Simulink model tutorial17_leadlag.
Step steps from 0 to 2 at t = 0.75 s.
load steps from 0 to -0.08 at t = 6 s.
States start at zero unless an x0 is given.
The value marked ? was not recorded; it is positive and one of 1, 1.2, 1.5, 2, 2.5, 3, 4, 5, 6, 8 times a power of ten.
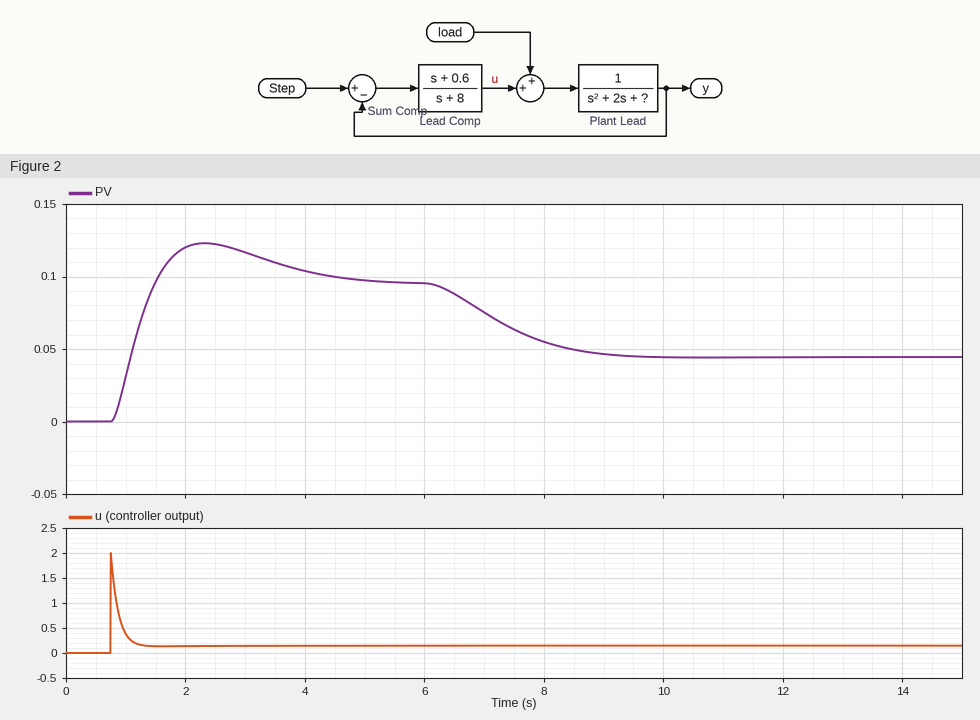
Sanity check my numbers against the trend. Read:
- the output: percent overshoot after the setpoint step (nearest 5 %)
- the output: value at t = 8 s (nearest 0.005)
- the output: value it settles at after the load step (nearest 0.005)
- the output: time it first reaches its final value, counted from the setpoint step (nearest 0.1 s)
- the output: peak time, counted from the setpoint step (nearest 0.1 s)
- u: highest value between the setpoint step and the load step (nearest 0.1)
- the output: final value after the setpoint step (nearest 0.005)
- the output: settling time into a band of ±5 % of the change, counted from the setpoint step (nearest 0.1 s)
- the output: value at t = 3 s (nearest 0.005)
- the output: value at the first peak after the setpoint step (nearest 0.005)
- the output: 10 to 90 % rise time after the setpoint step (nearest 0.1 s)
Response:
30 %
0.055
0.045
0.7 s
1.6 s
2.0
0.095
3.7 s
0.115
0.125
0.5 s
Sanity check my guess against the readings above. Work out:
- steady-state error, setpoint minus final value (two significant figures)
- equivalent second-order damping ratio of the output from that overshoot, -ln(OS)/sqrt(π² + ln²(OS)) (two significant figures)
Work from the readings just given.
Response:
1.9
0.36
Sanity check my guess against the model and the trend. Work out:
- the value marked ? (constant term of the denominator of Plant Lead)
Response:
1.5
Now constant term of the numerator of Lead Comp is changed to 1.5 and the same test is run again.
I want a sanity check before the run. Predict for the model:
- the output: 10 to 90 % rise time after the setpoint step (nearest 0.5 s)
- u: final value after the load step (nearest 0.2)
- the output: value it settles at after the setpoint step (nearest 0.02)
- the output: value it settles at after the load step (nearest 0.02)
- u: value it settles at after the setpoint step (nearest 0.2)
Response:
1.5 s
0.4
0.22
0.18
0.4
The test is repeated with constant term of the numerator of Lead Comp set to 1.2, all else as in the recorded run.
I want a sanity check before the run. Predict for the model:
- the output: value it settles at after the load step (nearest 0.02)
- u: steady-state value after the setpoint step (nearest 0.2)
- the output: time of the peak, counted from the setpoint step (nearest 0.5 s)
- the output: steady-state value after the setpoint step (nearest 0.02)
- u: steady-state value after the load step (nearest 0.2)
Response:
0.14
0.2
2.5 s
0.18
0.2
